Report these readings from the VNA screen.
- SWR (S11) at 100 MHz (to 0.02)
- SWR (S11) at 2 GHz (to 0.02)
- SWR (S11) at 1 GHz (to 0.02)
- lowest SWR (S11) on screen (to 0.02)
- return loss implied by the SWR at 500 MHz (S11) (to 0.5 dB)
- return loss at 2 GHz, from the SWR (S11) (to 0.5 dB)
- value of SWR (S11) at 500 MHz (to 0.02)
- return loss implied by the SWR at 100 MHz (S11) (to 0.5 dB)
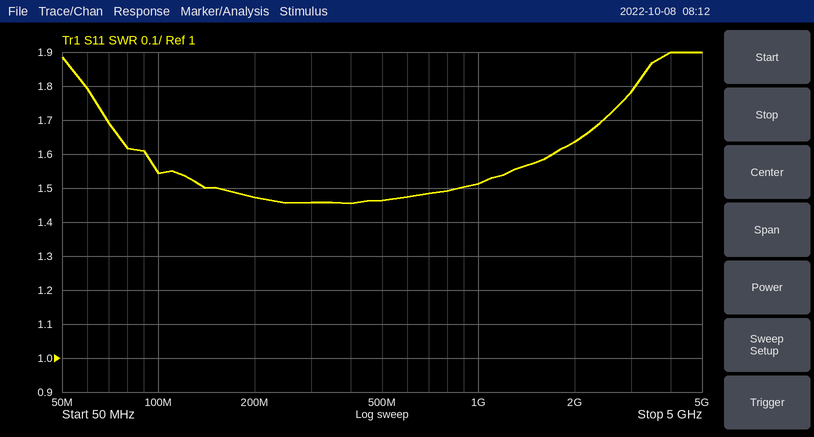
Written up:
1.54
1.64
1.52
1.46
14.5 dB
12.5 dB
1.46
13.5 dB
